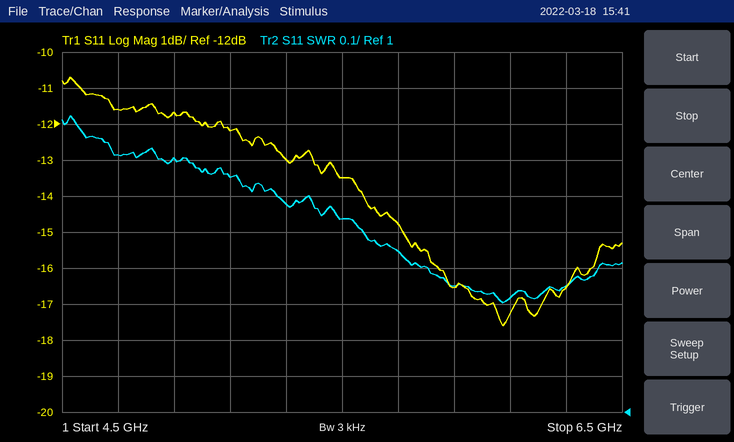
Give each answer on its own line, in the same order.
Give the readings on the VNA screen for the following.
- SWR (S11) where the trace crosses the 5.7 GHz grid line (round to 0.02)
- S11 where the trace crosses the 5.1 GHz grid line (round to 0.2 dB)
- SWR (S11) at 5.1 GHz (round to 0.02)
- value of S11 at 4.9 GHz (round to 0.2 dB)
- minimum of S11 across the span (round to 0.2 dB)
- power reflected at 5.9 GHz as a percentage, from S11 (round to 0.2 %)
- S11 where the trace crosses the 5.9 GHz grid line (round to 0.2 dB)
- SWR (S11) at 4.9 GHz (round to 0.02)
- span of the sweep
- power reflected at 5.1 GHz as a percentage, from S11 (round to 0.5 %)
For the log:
1.44
-12.2 dB
1.66
-11.6 dB
-17.6 dB
2.2 %
-16.6 dB
1.70
2 GHz
6.0 %
